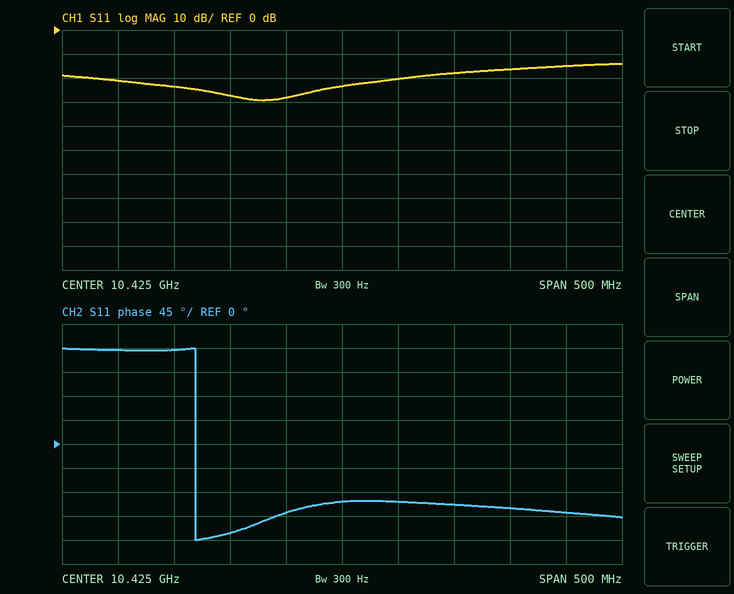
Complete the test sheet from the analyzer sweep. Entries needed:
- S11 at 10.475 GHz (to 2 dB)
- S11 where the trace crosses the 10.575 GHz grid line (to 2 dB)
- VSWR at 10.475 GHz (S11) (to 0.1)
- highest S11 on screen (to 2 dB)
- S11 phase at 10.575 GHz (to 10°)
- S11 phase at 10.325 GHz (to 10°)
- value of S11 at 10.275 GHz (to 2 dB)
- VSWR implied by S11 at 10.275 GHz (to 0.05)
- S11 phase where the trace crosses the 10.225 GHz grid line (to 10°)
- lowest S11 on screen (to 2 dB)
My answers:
-20 dB
-16 dB
1.2
-14 dB
-120°
-170°
-24 dB
1.15
180°
-30 dB
